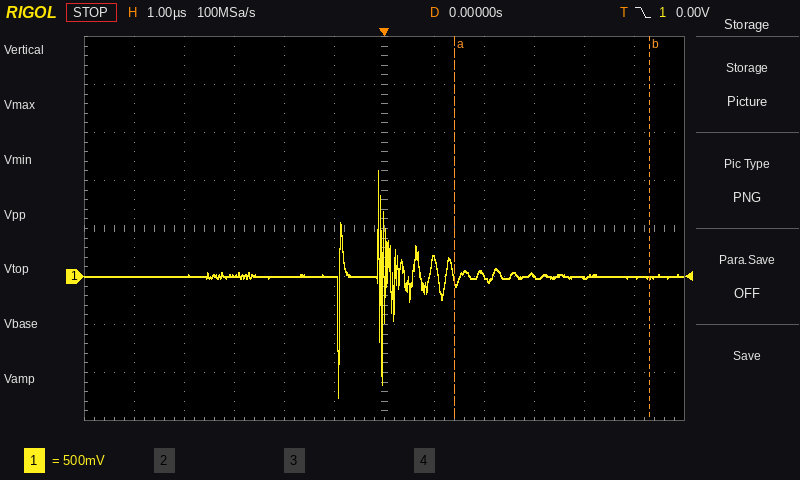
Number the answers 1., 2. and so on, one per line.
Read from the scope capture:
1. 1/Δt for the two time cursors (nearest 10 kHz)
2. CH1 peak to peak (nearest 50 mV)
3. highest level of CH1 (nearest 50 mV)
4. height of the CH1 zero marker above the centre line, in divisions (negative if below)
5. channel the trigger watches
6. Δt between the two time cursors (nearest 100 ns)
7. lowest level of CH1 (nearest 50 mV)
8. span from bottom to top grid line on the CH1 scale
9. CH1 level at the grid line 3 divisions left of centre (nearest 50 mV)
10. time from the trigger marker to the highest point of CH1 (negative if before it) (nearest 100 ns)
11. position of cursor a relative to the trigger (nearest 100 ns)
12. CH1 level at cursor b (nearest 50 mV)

1. 260 kHz
2. 2.35 V
3. 1.10 V
4. -1.0 div
5. CH1
6. 3.9 µs
7. -1.25 V
8. 4 V
9. 0 mV
10. -100 ns
11. +1.4 µs
12. 0 mV
